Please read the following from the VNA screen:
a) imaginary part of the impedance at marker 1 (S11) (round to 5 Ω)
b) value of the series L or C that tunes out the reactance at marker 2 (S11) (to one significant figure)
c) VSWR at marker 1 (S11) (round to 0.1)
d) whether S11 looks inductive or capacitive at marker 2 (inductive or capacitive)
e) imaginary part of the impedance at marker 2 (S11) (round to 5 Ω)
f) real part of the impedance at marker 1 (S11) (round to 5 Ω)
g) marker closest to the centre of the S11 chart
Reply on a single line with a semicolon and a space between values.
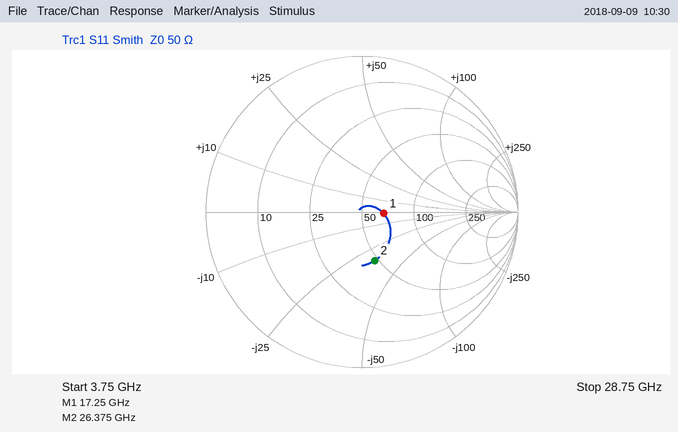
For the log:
0 Ω; 200 pH; 1.3; capacitive; -35 Ω; 65 Ω; marker 1
